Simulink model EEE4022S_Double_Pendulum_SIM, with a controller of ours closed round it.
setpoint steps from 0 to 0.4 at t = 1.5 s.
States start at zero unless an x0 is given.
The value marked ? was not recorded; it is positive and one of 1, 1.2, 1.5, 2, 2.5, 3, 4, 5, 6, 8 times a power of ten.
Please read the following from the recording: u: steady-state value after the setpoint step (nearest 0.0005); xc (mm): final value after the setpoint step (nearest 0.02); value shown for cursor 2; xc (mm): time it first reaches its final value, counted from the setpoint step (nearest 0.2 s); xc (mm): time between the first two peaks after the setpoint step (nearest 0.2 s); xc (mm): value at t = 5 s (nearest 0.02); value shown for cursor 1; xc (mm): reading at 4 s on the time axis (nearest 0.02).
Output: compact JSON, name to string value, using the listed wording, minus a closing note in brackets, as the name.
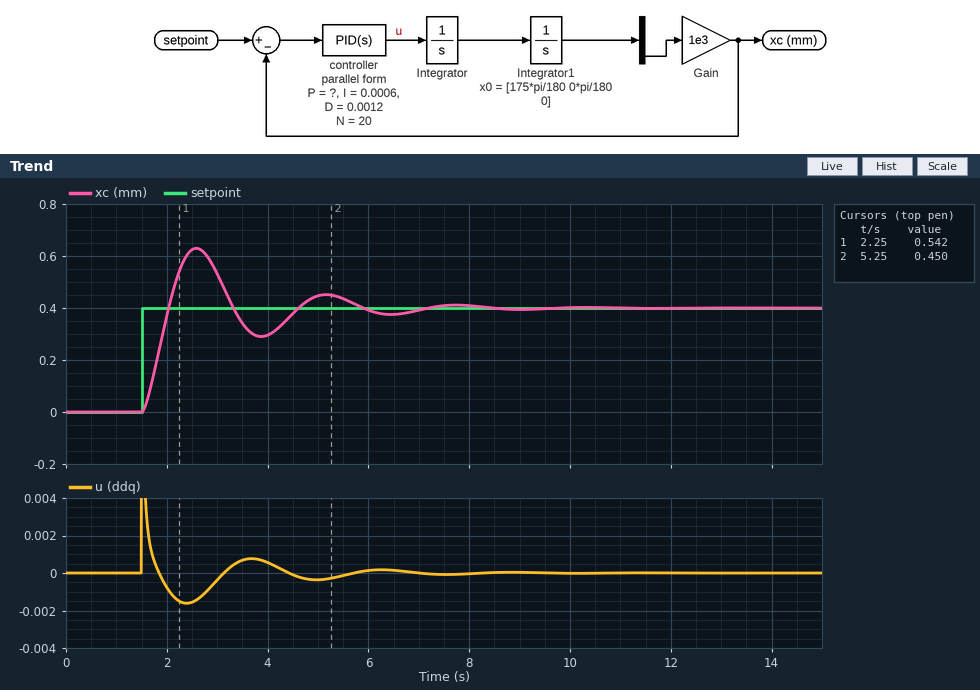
{"u: steady-state value after the setpoint step": "0.0000", "xc (mm): final value after the setpoint step": "0.40", "value shown for cursor 2": "0.450", "xc (mm): time it first reaches its final value, counted from the setpoint step": "0.6 s", "xc (mm): time between the first two peaks after the setpoint step": "2.6 s", "xc (mm): value at t = 5 s": "0.44", "value shown for cursor 1": "0.542", "xc (mm): reading at 4 s on the time axis": "0.30"}
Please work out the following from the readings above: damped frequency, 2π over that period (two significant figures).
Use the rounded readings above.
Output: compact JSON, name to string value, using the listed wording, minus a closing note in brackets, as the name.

{"damped frequency, 2π over that period": "2.4 rad/s"}
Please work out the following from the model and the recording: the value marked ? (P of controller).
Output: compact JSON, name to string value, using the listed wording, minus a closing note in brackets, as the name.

{"the value marked ?": "0.006"}
